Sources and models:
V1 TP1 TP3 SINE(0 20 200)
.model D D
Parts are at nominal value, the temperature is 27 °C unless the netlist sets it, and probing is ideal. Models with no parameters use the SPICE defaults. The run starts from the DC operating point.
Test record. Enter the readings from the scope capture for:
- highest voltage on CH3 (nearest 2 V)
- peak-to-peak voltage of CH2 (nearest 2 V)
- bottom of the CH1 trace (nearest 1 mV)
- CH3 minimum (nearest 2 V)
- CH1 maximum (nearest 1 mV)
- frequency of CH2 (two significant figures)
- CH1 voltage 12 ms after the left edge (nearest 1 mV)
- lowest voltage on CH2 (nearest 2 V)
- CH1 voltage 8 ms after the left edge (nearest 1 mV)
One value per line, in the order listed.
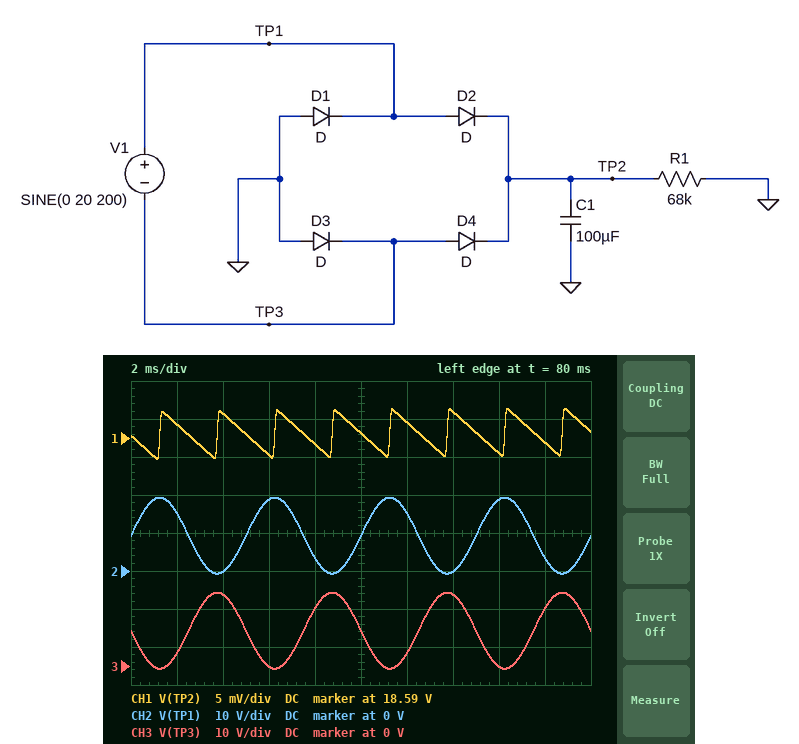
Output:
20 V
20 V
18.587 V
0 V
18.594 V
200 Hz
18.592 V
0 V
18.589 V
